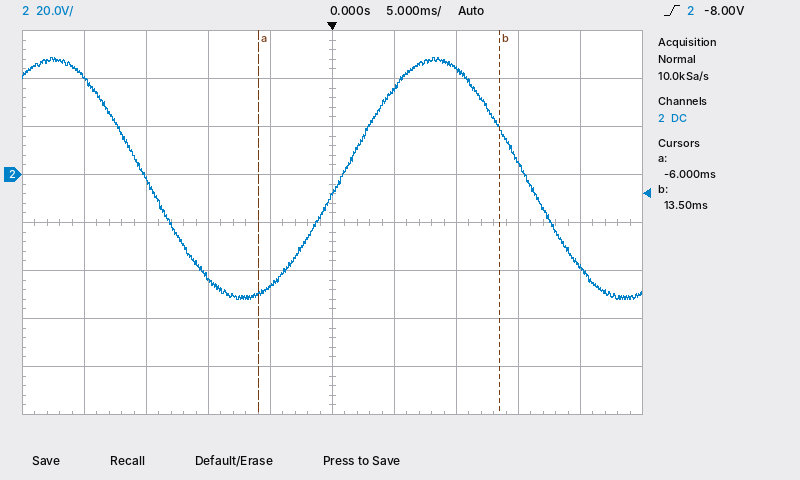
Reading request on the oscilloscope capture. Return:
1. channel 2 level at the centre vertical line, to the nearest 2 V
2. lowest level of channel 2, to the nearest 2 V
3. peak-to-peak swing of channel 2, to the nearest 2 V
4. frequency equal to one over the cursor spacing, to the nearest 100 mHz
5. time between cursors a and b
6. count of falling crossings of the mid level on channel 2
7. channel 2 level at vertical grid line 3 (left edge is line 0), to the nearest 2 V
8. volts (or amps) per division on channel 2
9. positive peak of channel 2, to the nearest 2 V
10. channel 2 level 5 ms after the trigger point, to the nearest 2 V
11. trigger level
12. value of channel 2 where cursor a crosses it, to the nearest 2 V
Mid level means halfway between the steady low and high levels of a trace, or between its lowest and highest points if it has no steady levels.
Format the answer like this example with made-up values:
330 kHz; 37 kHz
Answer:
-8 V; -52 V; 100 V; 51.3 Hz; 19.5 ms; 2; -42 V; 20 V; 48 V; 36 V; -8.00 V; -50 V
